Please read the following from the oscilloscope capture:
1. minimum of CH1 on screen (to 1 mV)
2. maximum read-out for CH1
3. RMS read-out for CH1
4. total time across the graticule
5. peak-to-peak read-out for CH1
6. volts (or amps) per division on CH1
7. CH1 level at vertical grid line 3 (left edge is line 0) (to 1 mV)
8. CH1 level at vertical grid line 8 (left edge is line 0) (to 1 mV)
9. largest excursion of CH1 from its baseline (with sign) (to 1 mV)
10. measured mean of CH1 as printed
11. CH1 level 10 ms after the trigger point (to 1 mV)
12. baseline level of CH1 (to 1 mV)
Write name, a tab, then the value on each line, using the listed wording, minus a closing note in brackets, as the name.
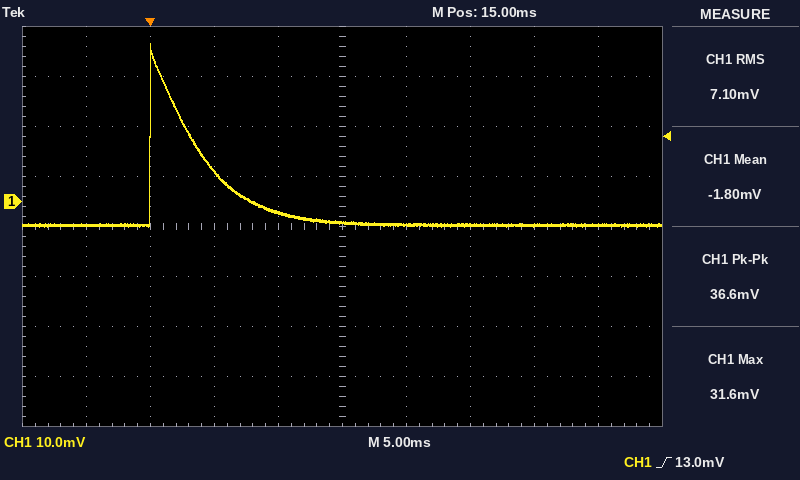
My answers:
minimum of CH1 on screen	-5 mV
maximum read-out for CH1	31.6 mV
RMS read-out for CH1	7.10 mV
total time across the graticule	50 ms
peak-to-peak read-out for CH1	36.6 mV
volts (or amps) per division on CH1	10 mV
CH1 level at vertical grid line 3 (left edge is line 0)	6 mV
CH1 level at vertical grid line 8 (left edge is line 0)	-5 mV
largest excursion of CH1 from its baseline (with sign)	+36 mV
measured mean of CH1 as printed	-1.80 mV
CH1 level 10 ms after the trigger point	-2 mV
baseline level of CH1	-5 mV
